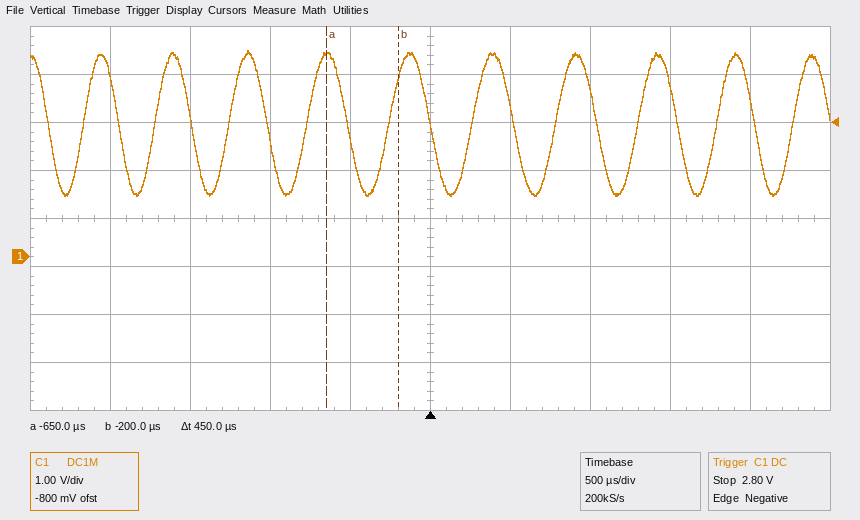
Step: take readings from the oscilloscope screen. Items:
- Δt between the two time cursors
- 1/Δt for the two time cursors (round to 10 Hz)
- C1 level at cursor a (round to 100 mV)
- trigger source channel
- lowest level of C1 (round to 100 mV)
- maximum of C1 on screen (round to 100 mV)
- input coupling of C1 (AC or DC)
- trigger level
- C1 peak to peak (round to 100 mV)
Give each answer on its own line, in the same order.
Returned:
450 µs
2.22 kHz
4.2 V
C1
1.3 V
4.3 V
DC
2.80 V
3.0 V
